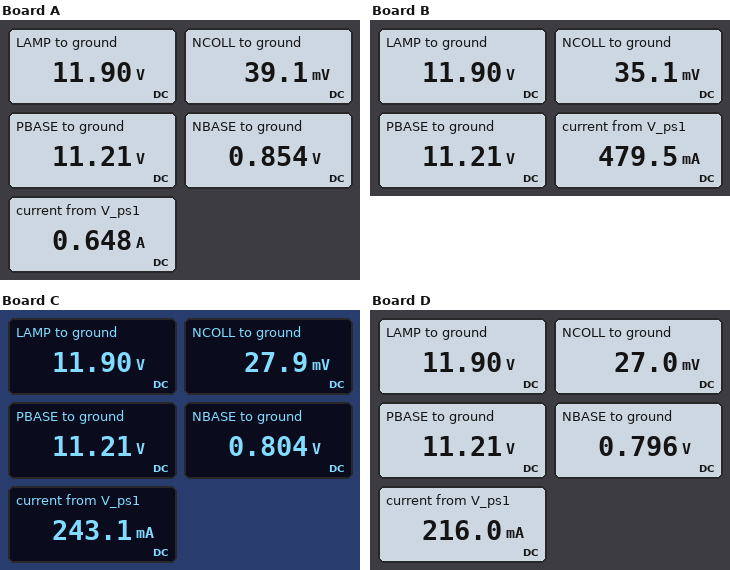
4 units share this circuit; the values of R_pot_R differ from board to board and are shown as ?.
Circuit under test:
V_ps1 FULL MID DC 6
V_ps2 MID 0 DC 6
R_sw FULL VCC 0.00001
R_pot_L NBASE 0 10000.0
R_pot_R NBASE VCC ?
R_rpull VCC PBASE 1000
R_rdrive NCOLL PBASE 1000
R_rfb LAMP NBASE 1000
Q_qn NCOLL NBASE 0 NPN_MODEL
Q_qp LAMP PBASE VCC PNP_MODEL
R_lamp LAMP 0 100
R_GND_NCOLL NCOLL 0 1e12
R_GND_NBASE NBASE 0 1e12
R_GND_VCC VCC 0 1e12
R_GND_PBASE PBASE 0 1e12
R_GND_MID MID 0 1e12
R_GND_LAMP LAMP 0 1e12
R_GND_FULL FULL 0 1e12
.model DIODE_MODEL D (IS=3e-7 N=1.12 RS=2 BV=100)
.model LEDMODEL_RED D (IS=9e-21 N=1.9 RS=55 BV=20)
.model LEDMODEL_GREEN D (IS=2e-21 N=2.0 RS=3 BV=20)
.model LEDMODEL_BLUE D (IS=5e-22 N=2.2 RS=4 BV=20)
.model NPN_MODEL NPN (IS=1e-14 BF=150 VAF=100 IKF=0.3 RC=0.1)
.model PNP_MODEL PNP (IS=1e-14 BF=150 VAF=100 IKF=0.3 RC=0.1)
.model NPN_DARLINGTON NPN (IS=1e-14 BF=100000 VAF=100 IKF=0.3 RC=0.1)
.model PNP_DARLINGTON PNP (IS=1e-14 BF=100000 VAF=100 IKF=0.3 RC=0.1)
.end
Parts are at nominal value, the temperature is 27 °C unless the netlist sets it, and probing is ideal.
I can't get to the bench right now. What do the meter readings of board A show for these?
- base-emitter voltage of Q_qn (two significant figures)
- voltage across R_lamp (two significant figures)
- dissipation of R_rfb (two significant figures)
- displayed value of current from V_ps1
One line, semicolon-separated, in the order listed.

850 mV; 12 V; 120 mW; 0.648 A
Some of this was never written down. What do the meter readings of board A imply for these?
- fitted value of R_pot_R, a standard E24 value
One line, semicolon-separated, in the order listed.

22 Ω
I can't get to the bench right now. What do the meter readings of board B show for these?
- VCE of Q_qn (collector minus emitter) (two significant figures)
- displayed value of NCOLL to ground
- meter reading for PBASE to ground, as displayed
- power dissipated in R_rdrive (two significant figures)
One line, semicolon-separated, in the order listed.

35 mV; 35.1 mV; 11.21 V; 120 mW
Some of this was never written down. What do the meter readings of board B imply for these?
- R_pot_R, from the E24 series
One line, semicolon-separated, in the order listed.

33 Ω
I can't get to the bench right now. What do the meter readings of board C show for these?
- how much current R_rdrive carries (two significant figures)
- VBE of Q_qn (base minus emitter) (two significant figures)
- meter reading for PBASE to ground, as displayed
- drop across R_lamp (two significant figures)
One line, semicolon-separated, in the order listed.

11 mA; 800 mV; 11.21 V; 12 V
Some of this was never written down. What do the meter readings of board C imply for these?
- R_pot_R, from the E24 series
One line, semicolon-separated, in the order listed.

110 Ω
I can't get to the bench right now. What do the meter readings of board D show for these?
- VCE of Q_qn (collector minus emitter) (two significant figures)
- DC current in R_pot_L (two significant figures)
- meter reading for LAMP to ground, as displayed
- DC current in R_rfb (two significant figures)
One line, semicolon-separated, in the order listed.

27 mV; 80 µA; 11.90 V; 11 mA
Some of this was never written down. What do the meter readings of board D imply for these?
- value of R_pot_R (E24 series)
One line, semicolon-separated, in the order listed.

150 Ω
